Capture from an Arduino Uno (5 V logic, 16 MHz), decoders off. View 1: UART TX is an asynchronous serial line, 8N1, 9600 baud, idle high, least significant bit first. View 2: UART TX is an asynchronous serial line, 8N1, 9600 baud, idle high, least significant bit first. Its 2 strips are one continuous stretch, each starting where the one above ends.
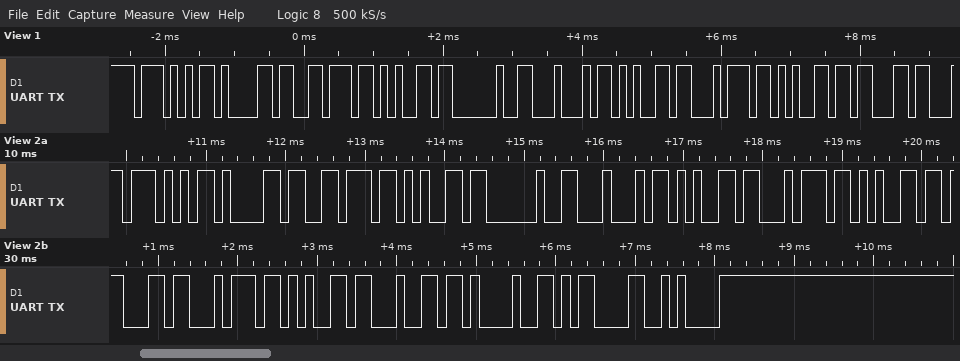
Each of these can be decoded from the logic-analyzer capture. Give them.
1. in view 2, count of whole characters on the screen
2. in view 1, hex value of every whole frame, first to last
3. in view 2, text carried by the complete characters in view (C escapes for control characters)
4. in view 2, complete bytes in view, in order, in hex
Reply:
16
57 61 76 65 20 44 65 74 65 63
"Wave Detected!\r\n"
57 61 76 65 20 44 65 74 65 63 74 65 64 21 0D 0A
